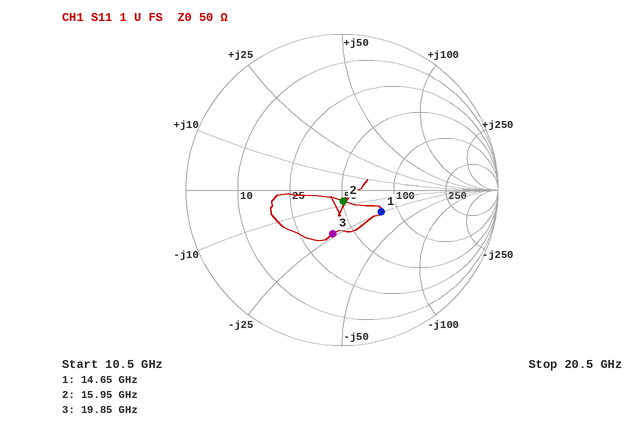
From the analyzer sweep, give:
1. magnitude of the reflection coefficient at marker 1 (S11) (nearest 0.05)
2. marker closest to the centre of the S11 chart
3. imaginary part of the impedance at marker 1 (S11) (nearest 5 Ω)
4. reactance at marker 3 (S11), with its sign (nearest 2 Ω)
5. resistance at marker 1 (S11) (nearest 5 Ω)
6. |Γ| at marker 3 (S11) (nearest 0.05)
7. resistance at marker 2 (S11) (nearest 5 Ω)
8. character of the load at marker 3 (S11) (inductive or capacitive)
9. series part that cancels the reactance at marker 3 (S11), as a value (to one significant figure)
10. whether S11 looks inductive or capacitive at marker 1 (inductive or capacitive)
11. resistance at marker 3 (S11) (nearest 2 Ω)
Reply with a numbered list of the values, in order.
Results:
1. 0.30
2. marker 2
3. -25 Ω
4. -24 Ω
5. 80 Ω
6. 0.30
7. 50 Ω
8. capacitive
9. 200 pH
10. capacitive
11. 38 Ω
